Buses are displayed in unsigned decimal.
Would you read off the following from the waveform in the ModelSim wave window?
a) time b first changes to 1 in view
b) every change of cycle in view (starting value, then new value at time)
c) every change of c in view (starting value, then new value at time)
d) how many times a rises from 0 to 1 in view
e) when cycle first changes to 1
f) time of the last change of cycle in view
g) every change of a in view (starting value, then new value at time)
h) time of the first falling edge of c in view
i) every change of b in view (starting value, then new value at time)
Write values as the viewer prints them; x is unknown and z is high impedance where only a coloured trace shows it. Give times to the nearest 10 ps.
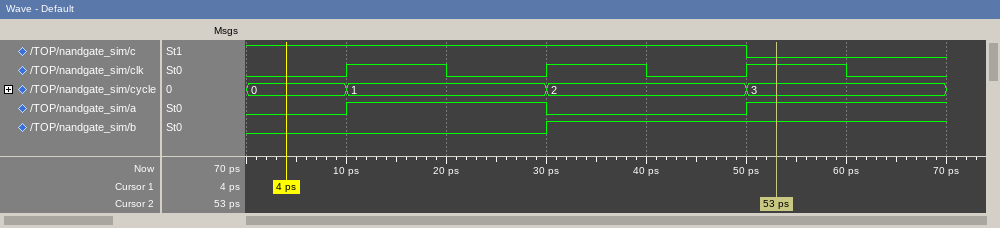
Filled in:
30 ps
0, 1 at 10 ps, 2 at 30 ps, 3 at 50 ps
1, 0 at 50 ps
2
10 ps
50 ps
0, 1 at 10 ps, 0 at 30 ps, 1 at 50 ps
50 ps
0, 1 at 30 ps
